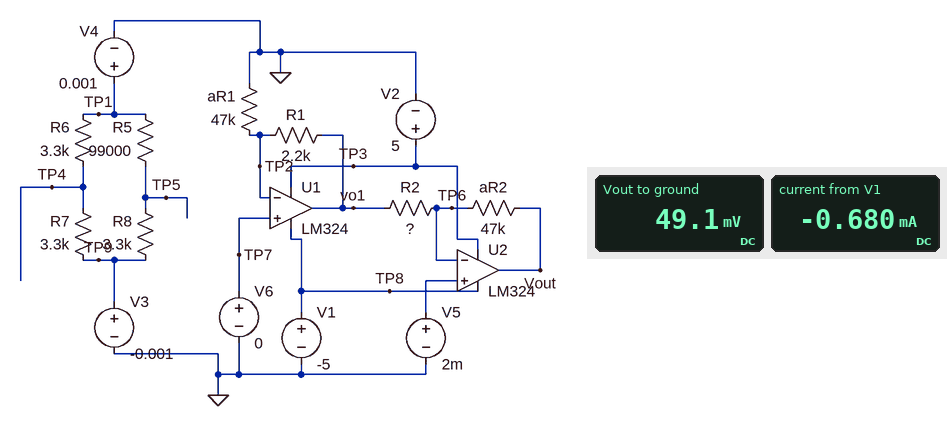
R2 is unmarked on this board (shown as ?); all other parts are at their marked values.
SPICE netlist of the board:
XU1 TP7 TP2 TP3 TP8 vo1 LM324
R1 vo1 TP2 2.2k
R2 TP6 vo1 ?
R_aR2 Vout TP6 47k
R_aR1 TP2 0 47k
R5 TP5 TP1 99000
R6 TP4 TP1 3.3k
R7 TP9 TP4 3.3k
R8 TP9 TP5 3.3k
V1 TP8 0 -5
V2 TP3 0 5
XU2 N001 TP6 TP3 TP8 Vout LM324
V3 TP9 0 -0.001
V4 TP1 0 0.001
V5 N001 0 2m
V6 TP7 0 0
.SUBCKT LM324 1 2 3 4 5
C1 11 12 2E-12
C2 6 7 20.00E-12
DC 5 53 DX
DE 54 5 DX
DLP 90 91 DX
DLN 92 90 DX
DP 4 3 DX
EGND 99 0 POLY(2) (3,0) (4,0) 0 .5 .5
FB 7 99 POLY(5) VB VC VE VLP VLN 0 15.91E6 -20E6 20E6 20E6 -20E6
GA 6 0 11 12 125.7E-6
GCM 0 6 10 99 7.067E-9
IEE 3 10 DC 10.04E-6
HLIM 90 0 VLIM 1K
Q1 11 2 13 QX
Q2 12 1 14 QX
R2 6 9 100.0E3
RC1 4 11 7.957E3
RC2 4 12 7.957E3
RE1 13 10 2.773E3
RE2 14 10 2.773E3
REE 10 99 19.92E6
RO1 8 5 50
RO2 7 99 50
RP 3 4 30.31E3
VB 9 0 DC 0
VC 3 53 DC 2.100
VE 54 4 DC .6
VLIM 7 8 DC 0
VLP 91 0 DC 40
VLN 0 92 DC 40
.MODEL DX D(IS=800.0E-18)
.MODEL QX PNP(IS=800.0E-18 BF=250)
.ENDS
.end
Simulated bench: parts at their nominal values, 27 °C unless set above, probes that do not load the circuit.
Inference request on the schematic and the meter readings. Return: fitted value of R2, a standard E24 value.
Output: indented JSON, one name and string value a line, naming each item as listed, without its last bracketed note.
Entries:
{
  "fitted value of R2, a standard E24 value": "2 kΩ"
}
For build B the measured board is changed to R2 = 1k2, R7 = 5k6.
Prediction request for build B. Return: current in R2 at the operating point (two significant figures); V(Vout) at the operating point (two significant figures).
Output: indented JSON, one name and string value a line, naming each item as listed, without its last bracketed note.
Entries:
{
  "current in R2 at the operating point": "1.7 µA",
  "V(Vout) at the operating point": "81 mV"
}
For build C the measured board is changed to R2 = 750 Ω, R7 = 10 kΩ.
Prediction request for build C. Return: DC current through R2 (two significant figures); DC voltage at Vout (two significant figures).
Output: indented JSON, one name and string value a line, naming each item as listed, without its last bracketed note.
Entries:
{
  "DC current through R2": "2.7 µA",
  "DC voltage at Vout": "130 mV"
}
